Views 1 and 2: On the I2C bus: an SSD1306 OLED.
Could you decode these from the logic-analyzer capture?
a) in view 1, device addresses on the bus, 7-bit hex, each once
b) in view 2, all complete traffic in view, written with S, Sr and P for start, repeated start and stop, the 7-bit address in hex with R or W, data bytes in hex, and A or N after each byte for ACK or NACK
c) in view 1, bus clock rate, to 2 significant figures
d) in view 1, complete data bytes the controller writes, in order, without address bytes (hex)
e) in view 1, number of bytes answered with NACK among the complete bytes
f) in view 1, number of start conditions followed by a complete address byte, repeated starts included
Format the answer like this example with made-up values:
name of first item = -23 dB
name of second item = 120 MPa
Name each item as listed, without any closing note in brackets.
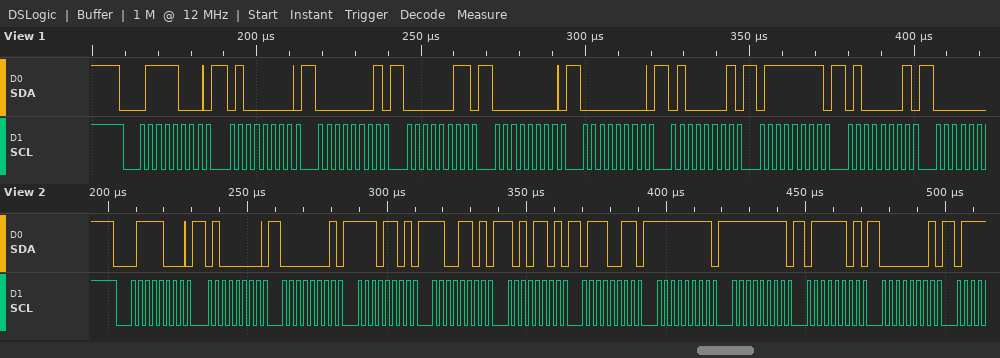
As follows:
in view 1, device addresses on the bus, 7-bit hex, each once = 0x3C
in view 2, all complete traffic in view, written with S, Sr and P for start, repeated start and stop, the 7-bit address in hex with R or W, data bytes in hex, and A or N after each byte for ACK or NACK = S 3CW A 40 A 01 A ED A CD A AD A 73 A FF A FF A 7D A 01 A
in view 1, bus clock rate, to 2 significant figures = 400 kHz
in view 1, complete data bytes the controller writes, in order, without address bytes = 40 01 03 00 00 41 7F 41
in view 1, number of bytes answered with NACK among the complete bytes = 0
in view 1, number of start conditions followed by a complete address byte, repeated starts included = 1
